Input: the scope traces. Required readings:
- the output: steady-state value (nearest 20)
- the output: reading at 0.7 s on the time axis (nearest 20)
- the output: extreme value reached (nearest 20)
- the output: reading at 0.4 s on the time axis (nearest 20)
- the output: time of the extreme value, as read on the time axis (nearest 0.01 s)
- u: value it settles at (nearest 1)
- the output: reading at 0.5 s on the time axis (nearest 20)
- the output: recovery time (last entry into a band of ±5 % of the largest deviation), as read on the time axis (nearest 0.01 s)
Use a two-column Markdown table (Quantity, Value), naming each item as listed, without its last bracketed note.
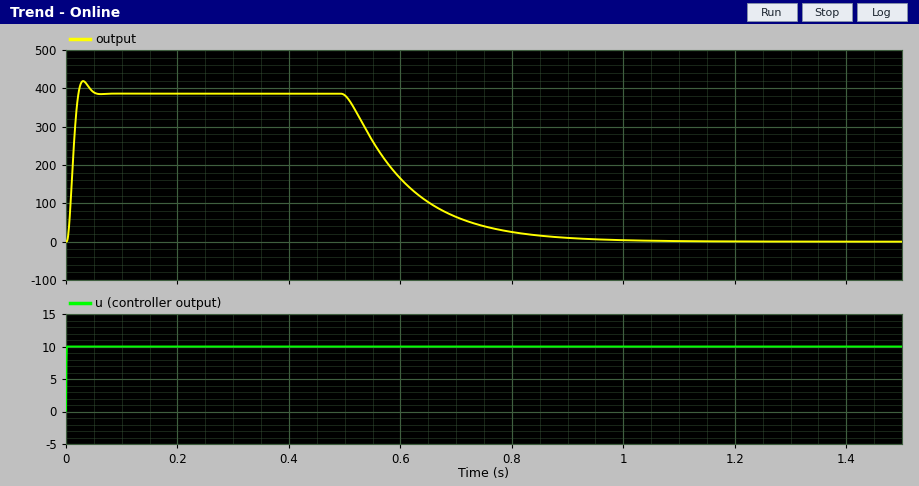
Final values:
| Quantity | Value |
|---|---|
| the output: steady-state value | 0 |
| the output: reading at 0.7 s on the time axis | 60 |
| the output: extreme value reached | 420 |
| the output: reading at 0.4 s on the time axis | 380 |
| the output: time of the extreme value, as read on the time axis | 0.03 s |
| u: value it settles at | 10 |
| the output: reading at 0.5 s on the time axis | 380 |
| the output: recovery time (last entry into a band of ±5 % of the largest deviation), as read on the time axis | 0.82 s |
